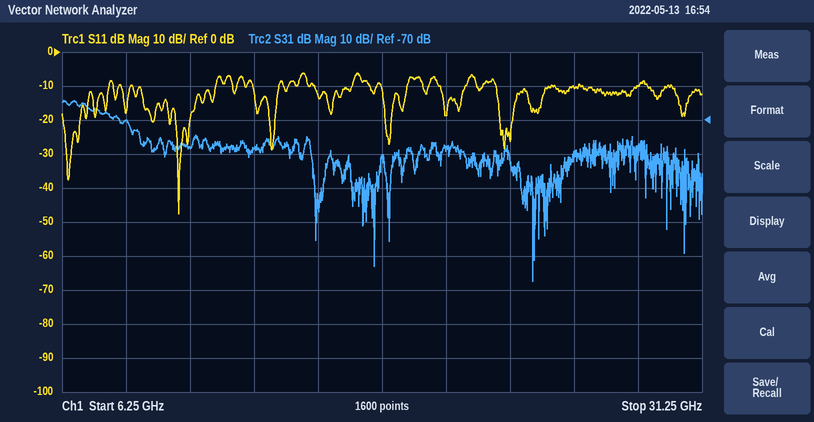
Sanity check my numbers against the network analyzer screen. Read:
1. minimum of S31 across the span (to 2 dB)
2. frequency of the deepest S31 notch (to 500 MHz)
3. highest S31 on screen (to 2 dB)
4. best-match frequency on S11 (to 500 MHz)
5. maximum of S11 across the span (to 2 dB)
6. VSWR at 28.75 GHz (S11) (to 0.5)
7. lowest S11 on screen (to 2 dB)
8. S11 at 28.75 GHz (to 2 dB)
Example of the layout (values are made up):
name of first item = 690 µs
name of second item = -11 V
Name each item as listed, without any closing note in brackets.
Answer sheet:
minimum of S31 across the span = -118 dB
frequency of the deepest S31 notch = 24.5 GHz
highest S31 on screen = -64 dB
best-match frequency on S11 = 11.0 GHz
maximum of S11 across the span = -6 dB
VSWR at 28.75 GHz (S11) = 2.0
lowest S11 on screen = -48 dB
S11 at 28.75 GHz = -10 dB
